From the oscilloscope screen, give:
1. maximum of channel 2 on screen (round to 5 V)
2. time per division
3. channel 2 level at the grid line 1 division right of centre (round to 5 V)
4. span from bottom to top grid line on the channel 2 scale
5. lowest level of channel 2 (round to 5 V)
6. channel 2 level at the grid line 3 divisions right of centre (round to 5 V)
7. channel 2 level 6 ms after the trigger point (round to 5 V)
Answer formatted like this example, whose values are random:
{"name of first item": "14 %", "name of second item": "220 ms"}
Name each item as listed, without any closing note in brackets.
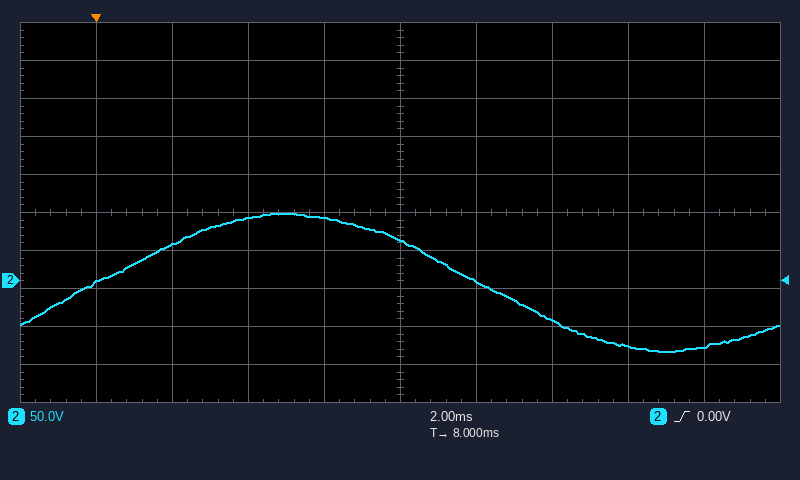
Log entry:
{"maximum of channel 2 on screen": "90 V", "time per division": "2 ms", "channel 2 level at the grid line 1 division right of centre": "0 V", "span from bottom to top grid line on the channel 2 scale": "500 V", "lowest level of channel 2": "-95 V", "channel 2 level at the grid line 3 divisions right of centre": "-85 V", "channel 2 level 6 ms after the trigger point": "85 V"}
